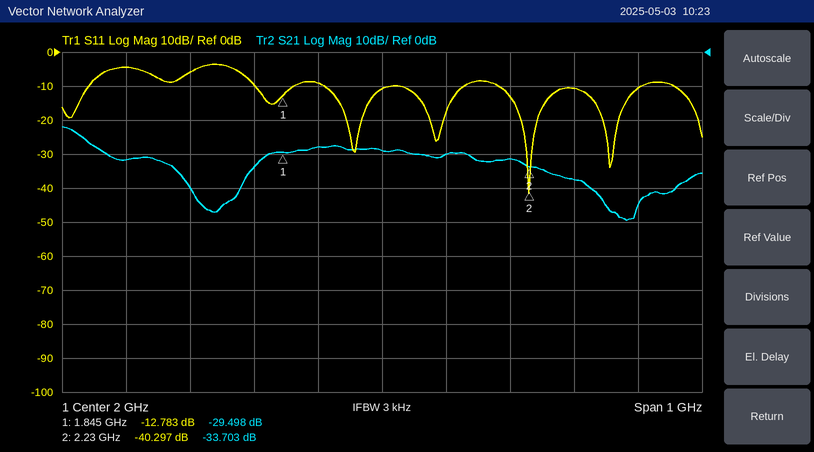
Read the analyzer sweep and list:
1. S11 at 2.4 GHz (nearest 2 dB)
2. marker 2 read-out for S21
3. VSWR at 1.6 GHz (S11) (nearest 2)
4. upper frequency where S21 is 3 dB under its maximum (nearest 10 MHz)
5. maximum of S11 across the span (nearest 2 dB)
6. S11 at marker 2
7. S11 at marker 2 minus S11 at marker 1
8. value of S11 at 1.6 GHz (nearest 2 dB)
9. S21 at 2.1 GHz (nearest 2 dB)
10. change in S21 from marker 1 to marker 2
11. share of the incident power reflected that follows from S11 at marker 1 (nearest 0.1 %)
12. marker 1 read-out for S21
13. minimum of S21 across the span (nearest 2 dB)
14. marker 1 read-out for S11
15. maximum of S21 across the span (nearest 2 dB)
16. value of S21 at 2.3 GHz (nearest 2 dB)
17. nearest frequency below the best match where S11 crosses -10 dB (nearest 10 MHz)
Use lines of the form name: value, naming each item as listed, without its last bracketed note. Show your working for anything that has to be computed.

S11 at 2.4 GHz: -10 dB
marker 2 read-out for S21: -33.703 dB
VSWR at 1.6 GHz (S11): |Γ| = 10^(-4/20) = 0.6310; VSWR = (1 + 0.6310)/(1 − 0.6310) ≈ 4
upper frequency where S21 is 3 dB under its maximum: 1.53 GHz
maximum of S11 across the span: -4 dB
S11 at marker 2: -40.297 dB
S11 at marker 2 minus S11 at marker 1: -40.297 − (-12.783) = -27.514 dB
value of S11 at 1.6 GHz: -4 dB
S21 at 2.1 GHz: -30 dB
change in S21 from marker 1 to marker 2: -33.703 − (-29.498) = -4.205 dB
share of the incident power reflected that follows from S11 at marker 1: 10^(-12.783/10) ≈ 5.3 %
marker 1 read-out for S21: -29.498 dB
minimum of S21 across the span: -50 dB
marker 1 read-out for S11: -12.783 dB
maximum of S21 across the span: -22 dB
value of S21 at 2.3 GHz: -38 dB
nearest frequency below the best match where S11 crosses -10 dB: 2.18 GHz
